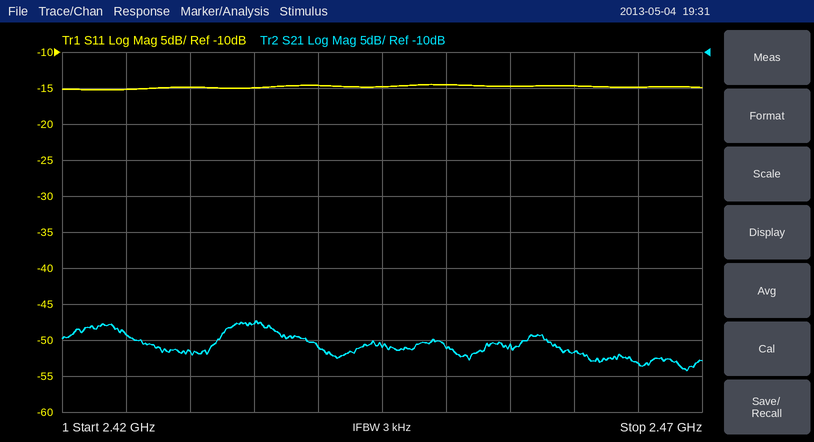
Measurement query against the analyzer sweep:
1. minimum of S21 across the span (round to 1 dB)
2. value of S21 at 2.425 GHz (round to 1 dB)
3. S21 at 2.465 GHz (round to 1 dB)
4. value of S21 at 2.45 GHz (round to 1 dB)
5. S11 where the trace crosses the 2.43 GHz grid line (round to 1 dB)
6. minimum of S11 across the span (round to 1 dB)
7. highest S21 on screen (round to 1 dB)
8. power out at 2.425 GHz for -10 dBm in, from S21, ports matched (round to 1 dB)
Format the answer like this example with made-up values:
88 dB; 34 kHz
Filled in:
-54 dB; -49 dB; -53 dB; -51 dB; -15 dB; -15 dB; -47 dB; -59 dBm
